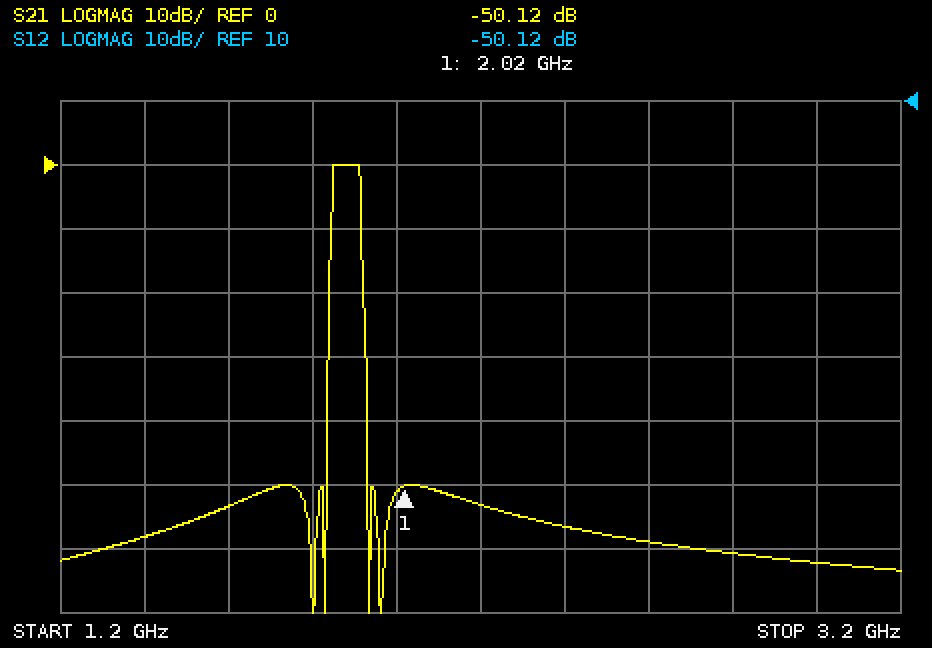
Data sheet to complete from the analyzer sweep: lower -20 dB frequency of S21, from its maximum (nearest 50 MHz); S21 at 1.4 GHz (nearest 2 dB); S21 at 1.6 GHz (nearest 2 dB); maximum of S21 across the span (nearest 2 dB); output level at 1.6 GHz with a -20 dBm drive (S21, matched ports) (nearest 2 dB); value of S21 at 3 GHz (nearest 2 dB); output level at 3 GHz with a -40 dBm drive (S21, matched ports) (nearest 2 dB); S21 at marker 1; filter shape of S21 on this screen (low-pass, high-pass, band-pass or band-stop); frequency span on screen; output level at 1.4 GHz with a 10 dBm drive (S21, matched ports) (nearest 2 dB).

1.85 GHz
-58 dB
-54 dB
0 dB
-74 dBm
-62 dB
-102 dBm
-50.12 dB
band-pass
2 GHz
-48 dBm
